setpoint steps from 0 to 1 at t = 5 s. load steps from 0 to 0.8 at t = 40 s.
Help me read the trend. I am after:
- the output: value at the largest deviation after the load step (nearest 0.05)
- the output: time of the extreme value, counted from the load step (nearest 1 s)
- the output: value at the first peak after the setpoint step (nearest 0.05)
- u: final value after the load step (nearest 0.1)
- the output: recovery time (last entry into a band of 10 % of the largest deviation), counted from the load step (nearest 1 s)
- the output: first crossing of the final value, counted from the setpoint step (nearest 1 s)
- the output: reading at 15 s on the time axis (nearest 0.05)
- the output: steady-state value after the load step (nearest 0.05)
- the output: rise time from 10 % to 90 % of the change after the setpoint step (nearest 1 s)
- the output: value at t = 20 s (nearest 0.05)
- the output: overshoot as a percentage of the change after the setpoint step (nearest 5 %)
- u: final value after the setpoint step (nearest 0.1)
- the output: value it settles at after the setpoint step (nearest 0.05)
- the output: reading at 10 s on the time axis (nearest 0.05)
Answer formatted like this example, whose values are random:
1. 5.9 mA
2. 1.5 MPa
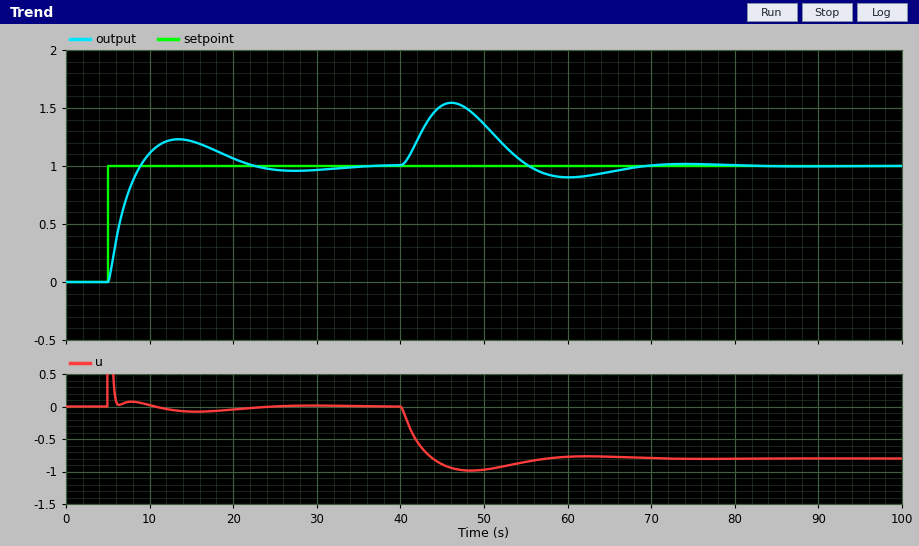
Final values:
1. 1.55
2. 6 s
3. 1.25
4. -0.8
5. 25 s
6. 4 s
7. 1.20
8. 1.00
9. 3 s
10. 1.05
11. 25 %
12. 0.0
13. 1.00
14. 1.10
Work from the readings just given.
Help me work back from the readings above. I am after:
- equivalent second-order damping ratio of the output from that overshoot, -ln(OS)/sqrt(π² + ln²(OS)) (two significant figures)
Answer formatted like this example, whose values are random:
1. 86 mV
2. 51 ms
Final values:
1. 0.40
